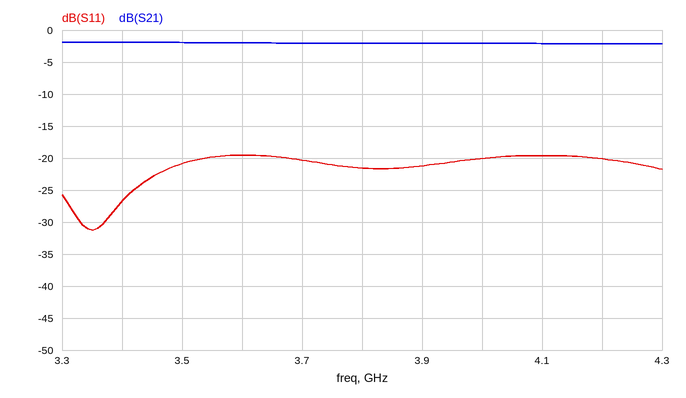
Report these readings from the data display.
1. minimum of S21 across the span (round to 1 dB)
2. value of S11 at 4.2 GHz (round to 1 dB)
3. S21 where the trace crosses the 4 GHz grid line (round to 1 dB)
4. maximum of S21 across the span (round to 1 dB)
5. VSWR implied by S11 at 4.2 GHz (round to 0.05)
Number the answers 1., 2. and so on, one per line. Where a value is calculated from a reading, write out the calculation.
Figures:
1. -2 dB
2. -20 dB
3. -2 dB
4. -2 dB
5. |Γ| = 10^(-20/20) = 0.1000; VSWR = (1 + 0.1000)/(1 − 0.1000) ≈ 1.22, so 1.20 to the nearest 0.05
